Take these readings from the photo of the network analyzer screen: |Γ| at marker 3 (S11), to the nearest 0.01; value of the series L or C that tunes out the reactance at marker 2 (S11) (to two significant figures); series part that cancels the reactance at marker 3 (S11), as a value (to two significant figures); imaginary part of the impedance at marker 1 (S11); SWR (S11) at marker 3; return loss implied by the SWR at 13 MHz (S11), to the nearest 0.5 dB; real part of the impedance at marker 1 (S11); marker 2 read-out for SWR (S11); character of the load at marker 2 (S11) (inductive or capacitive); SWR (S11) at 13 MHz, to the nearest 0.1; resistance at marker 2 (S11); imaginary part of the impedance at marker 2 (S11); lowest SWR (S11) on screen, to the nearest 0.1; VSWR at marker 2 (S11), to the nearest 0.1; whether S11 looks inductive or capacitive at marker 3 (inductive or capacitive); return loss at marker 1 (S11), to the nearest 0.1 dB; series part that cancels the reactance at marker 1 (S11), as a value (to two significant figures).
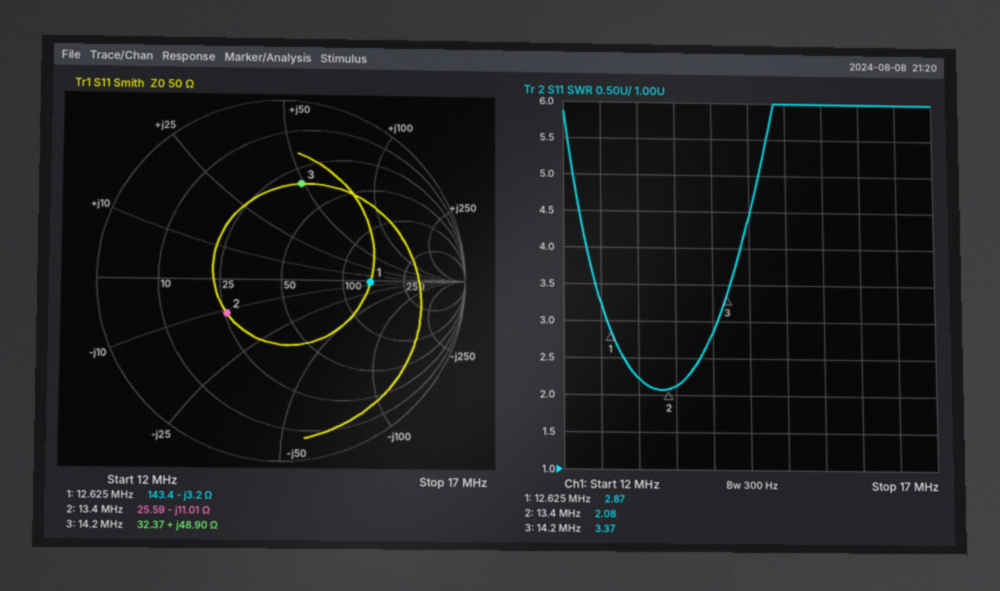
0.54
130 nH
230 pF
-3.2 Ω
3.37
8.5 dB
143.4 Ω
2.08
capacitive
2.2
25.59 Ω
-11.01 Ω
2.1
2.1
inductive
6.3 dB
40 nH
